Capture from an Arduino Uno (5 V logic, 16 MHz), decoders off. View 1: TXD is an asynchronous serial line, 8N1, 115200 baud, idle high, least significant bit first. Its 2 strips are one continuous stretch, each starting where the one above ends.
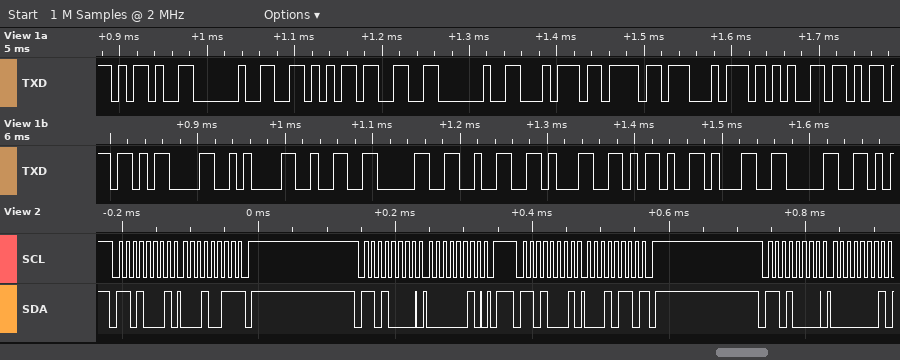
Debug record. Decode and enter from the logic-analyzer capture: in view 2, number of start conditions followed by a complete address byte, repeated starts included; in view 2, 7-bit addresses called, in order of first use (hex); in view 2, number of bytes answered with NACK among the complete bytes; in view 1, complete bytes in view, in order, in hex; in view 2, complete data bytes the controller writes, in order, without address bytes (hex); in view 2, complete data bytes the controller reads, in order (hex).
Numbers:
4
0x68
2
2D 20 56 33 20 74 6F 74 65 6D 0D 0A 32 30 32 31 2D 31 30
02 01
13 16
